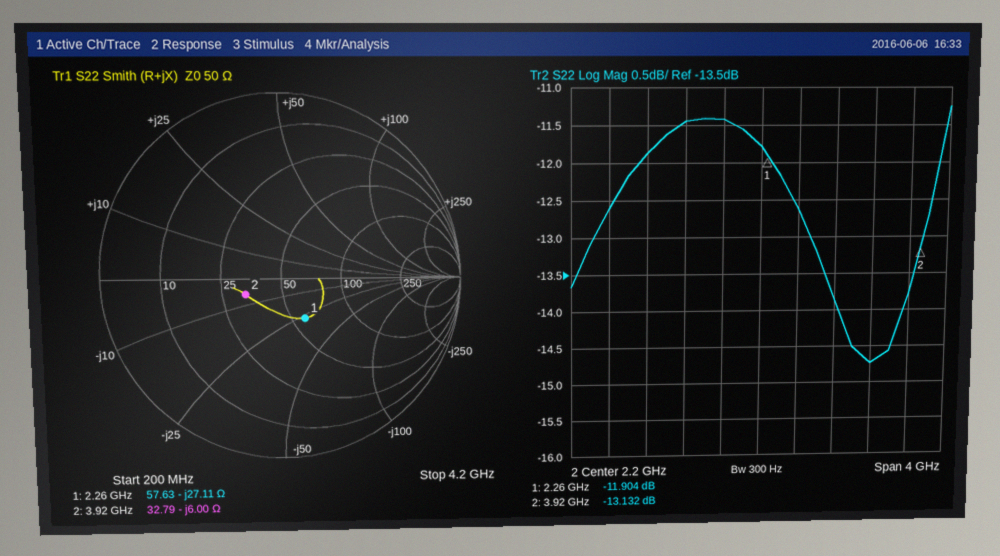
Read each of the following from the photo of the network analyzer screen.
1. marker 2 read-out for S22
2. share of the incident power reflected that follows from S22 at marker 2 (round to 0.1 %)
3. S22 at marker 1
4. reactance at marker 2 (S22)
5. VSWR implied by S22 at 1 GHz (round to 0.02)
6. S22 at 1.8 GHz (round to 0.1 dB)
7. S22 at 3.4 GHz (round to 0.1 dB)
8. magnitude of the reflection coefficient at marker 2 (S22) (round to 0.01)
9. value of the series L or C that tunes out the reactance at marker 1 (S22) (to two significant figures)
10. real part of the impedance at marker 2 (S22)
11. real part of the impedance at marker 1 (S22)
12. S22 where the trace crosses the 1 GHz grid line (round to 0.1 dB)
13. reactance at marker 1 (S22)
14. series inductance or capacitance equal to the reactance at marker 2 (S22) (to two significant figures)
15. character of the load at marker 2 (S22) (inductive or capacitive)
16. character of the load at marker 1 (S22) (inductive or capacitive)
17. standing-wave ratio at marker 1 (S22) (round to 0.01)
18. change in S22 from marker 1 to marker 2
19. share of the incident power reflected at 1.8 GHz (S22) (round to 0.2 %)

-13.132 dB
4.9 %
-11.904 dB
-6.00 Ω
1.68
-11.4 dB
-14.7 dB
0.22
1.9 nH
32.79 Ω
57.63 Ω
-11.9 dB
-27.11 Ω
6.8 pF
capacitive
capacitive
1.68
-1.228 dB
7.2 %
